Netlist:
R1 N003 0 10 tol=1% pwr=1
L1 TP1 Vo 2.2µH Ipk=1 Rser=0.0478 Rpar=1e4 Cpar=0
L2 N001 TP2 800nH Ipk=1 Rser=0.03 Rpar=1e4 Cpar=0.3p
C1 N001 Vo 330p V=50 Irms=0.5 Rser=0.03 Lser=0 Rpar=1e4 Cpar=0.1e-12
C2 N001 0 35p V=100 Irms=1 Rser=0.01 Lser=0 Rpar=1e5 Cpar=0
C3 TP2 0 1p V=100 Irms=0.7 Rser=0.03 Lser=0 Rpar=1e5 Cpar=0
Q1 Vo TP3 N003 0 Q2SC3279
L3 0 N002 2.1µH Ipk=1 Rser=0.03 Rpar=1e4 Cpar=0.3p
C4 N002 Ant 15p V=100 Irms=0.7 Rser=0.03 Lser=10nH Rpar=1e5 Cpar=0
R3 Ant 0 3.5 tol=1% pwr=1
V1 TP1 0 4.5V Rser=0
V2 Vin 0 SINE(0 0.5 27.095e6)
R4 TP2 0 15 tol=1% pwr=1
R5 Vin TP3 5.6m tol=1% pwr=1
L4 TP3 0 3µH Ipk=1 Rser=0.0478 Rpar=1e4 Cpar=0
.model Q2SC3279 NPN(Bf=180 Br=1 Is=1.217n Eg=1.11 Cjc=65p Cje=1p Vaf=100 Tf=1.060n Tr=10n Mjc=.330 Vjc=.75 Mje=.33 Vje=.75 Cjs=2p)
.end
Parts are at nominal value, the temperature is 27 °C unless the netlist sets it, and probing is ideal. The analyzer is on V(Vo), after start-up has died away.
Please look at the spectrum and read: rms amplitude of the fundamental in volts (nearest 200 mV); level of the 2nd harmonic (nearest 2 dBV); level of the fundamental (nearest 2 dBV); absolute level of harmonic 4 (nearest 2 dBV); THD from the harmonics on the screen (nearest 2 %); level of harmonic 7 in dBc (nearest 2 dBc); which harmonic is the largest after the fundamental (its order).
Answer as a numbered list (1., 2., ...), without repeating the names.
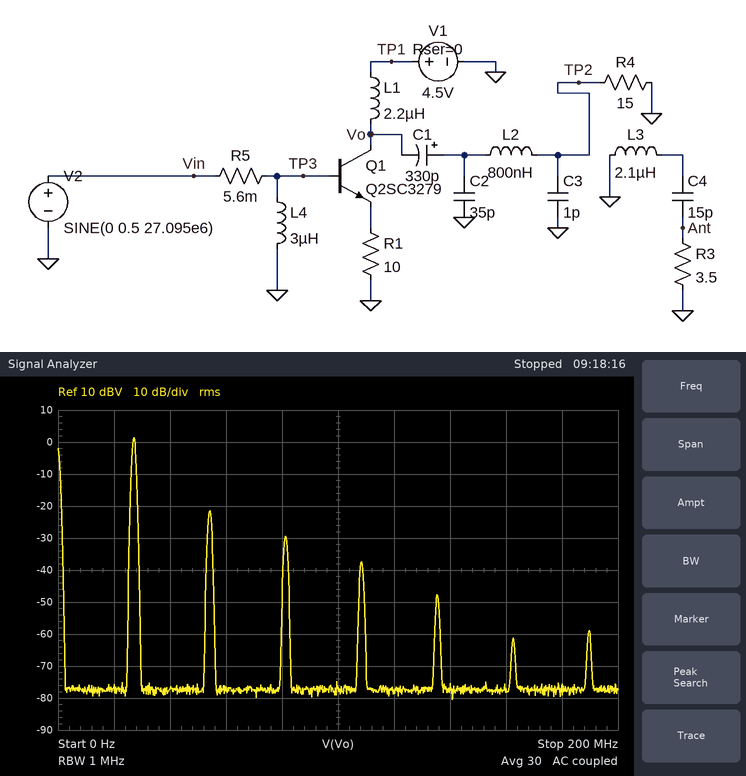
1. 1.2 V
2. -22 dBV
3. 2 dBV
4. -38 dBV
5. 8 %
6. -60 dBc
7. 2
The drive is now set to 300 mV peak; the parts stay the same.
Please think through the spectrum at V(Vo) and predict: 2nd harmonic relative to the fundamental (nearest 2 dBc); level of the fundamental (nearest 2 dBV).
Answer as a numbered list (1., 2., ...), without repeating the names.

1. -46 dBc
2. -6 dBV
